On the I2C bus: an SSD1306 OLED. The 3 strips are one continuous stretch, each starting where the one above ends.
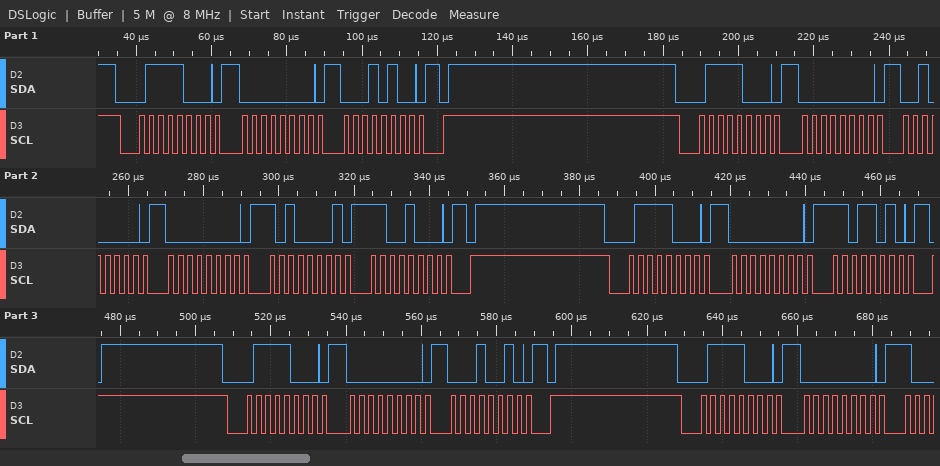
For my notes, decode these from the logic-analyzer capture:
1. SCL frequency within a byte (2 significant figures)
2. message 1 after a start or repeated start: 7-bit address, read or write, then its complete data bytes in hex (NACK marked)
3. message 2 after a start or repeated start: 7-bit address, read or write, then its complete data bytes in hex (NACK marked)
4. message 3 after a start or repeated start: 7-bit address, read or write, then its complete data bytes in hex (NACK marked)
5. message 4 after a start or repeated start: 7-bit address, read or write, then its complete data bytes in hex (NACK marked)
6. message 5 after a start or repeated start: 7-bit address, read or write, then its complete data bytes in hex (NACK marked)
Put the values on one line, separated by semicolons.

400 kHz; 0x3C write: 00 14; 0x3C write: 00 20 00 A1 C8; 0x3C write: 00 DA; 0x3C write: 00 12; 0x3C write: 00
